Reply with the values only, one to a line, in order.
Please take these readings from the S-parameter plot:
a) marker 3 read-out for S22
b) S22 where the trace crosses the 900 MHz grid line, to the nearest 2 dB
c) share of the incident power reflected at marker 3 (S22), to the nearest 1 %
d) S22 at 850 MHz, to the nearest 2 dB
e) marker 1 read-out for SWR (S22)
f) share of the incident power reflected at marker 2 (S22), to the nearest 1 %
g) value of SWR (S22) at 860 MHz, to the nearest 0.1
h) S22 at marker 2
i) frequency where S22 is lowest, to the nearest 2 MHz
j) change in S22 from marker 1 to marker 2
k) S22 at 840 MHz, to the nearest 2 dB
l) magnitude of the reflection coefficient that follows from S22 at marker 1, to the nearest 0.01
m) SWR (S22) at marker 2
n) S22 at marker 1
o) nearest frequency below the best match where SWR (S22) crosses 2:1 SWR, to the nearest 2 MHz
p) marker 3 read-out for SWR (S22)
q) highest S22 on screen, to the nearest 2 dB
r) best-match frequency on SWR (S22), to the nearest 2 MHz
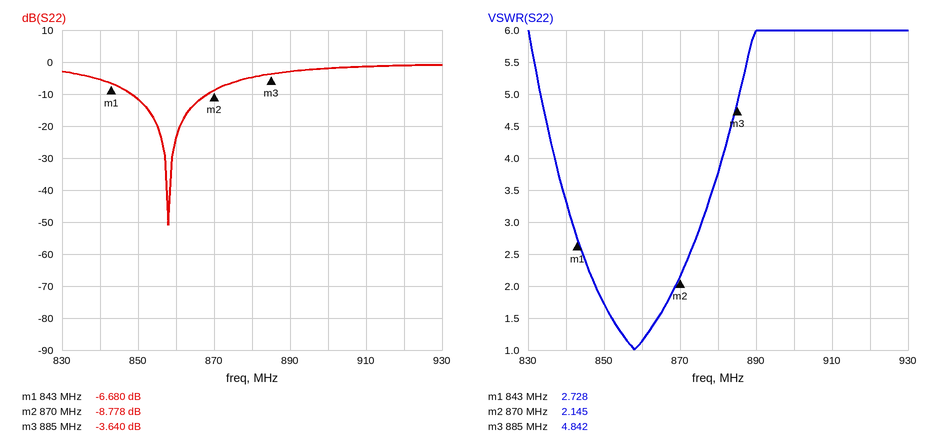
-3.640 dB
-2 dB
43 %
-12 dB
2.728
13 %
1.1
-8.778 dB
858 MHz
-2.098 dB
-6 dB
0.46
2.145
-6.680 dB
848 MHz
4.842
0 dB
858 MHz
